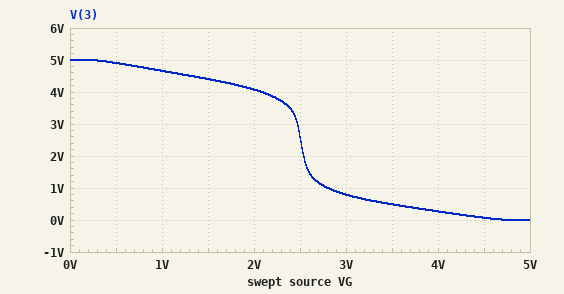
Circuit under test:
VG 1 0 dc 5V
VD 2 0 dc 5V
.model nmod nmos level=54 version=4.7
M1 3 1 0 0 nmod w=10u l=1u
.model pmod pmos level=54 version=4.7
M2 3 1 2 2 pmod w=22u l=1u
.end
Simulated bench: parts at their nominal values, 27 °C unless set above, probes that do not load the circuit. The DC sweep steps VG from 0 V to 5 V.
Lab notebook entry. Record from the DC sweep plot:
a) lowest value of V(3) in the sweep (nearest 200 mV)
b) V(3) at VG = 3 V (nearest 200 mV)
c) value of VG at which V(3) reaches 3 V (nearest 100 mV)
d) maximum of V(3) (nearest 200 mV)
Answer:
0 V
800 mV
2.5 V
5.0 V
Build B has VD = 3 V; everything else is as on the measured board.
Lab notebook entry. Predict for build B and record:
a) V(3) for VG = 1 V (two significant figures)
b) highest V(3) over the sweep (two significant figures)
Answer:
2.7 V
3.0 V
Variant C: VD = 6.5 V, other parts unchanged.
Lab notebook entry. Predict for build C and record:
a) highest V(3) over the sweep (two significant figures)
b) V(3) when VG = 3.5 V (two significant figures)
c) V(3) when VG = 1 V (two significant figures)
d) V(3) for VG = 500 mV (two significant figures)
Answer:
6.5 V
1.8 V
5.9 V
6.3 V
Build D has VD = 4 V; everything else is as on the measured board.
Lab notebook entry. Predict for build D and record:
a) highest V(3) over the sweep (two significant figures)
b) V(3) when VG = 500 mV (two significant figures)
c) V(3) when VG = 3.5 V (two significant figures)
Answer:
4.0 V
3.9 V
44 mV
